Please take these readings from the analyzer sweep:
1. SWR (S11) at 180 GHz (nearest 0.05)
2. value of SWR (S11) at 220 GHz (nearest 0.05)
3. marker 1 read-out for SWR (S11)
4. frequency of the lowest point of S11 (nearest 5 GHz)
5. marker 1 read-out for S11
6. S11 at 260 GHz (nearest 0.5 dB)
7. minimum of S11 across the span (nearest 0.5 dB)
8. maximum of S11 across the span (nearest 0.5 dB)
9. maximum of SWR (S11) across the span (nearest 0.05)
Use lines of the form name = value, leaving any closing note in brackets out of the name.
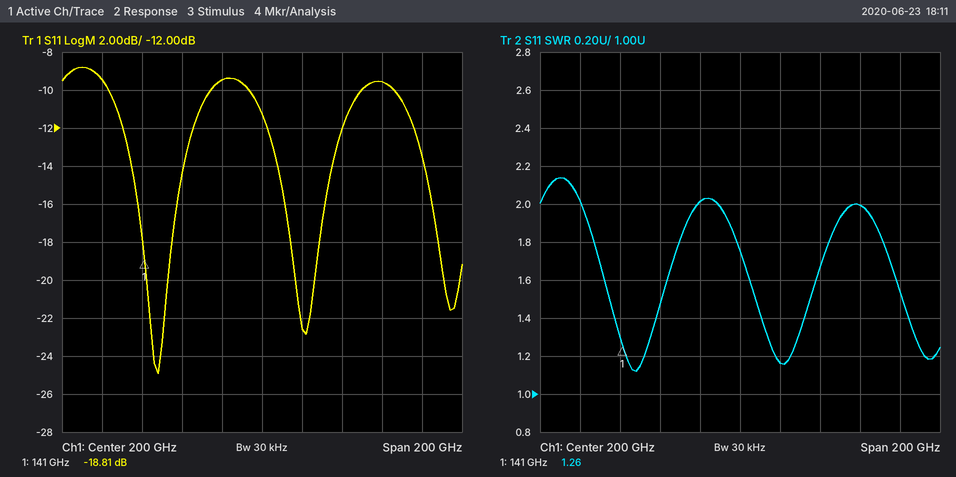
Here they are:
SWR (S11) at 180 GHz = 2.00
value of SWR (S11) at 220 GHz = 1.15
marker 1 read-out for SWR = 1.26
frequency of the lowest point of S11 = 150 GHz
marker 1 read-out for S11 = -18.81 dB
S11 at 260 GHz = -9.5 dB
minimum of S11 across the span = -25.0 dB
maximum of S11 across the span = -9.0 dB
maximum of SWR (S11) across the span = 2.15
